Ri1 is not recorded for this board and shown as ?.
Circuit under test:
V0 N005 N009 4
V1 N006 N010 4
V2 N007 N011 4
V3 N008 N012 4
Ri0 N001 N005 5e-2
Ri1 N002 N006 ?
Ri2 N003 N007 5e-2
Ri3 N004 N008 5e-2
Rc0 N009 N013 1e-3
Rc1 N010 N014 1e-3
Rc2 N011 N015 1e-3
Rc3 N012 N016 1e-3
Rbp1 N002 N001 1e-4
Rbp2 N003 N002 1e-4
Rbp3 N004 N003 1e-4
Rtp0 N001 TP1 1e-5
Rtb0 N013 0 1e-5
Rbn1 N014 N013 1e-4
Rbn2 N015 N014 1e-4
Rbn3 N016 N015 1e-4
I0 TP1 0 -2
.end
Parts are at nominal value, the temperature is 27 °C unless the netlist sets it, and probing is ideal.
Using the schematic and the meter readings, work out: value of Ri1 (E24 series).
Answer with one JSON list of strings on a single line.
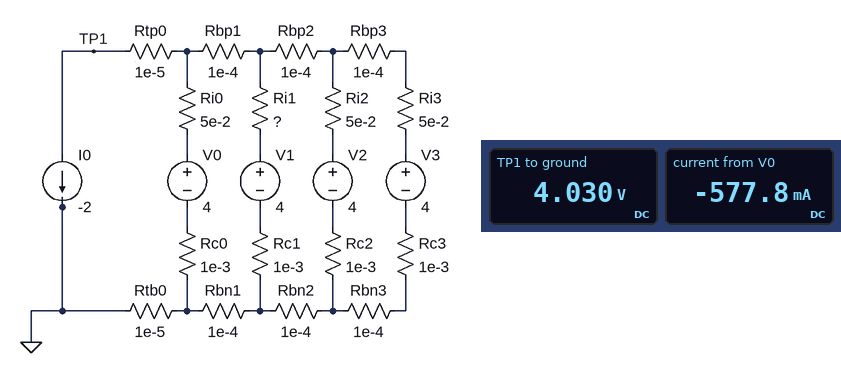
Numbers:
["0.1 Ω"]
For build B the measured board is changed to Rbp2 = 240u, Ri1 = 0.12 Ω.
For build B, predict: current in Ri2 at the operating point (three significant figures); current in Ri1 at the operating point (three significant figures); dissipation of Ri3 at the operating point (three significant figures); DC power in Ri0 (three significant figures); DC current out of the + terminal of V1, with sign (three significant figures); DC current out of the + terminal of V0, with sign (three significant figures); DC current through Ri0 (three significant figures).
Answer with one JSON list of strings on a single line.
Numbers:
["580 mA", "248 mA", "16.7 mW", "17.6 mW", "-248 mA", "-594 mA", "594 mA"]
